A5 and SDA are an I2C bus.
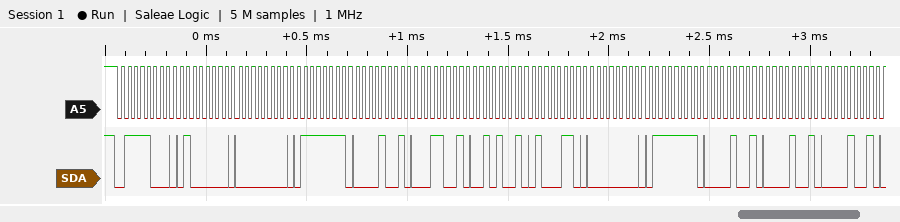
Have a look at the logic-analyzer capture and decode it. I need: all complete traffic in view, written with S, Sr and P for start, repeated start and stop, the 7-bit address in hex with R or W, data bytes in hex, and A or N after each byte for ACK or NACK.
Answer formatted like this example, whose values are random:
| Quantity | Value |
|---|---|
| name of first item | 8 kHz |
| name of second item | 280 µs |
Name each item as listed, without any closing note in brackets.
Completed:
| Quantity | Value |
|---|---|
| all complete traffic in view, written with S, Sr and P for start, repeated start and stop, the 7-bit address in hex with R or W, data bytes in hex, and A or N after each byte for ACK or NACK | S 3CW A 40 A 00 A 7F A 09 A 19 A 29 A 46 A 00 A 7F A 09 A 09 A 09 A |
